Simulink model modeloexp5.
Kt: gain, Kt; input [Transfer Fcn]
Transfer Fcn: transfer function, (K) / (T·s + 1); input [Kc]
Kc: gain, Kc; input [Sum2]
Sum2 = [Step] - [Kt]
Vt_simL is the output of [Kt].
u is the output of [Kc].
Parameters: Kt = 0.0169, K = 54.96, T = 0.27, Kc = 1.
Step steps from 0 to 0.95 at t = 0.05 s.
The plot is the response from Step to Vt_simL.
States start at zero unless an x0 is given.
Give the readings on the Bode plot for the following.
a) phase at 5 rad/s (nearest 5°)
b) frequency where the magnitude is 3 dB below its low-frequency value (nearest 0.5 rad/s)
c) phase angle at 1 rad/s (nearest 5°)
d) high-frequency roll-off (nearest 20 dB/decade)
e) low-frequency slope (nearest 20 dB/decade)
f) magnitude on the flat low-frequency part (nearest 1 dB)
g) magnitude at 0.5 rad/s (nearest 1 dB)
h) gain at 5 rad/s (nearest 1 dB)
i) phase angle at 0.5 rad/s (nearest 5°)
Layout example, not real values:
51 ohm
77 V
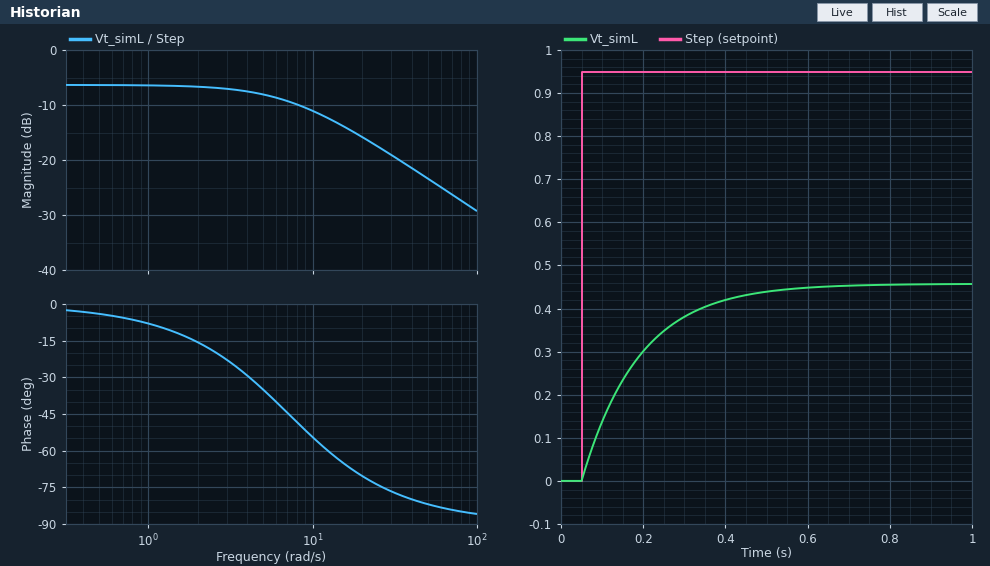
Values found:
-35°
7.0 rad/s
-10°
-20 dB/decade
0 dB/decade
-6 dB
-6 dB
-8 dB
-5°
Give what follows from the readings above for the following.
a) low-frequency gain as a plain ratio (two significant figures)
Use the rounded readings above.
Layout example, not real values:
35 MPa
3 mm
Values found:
0.50
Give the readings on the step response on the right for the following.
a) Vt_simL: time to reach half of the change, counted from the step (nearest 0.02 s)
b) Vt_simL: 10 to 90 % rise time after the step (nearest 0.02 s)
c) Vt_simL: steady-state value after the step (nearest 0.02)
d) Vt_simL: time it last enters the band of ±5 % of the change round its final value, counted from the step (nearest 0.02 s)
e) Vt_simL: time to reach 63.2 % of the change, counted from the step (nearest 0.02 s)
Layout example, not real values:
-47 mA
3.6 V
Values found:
0.10 s
0.30 s
0.46
0.42 s
0.14 s
